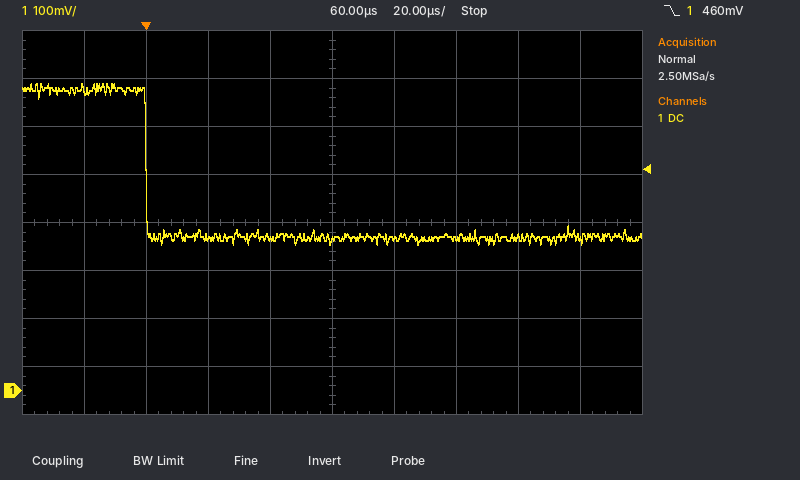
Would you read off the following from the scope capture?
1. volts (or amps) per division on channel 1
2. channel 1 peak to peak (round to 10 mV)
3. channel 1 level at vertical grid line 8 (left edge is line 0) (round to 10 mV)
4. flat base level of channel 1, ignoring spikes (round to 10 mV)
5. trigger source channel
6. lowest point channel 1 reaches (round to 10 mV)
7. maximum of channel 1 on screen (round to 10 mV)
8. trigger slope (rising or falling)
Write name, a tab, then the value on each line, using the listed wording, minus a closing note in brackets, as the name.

volts (or amps) per division on channel 1	100 mV
channel 1 peak to peak	340 mV
channel 1 level at vertical grid line 8 (left edge is line 0)	320 mV
flat base level of channel 1, ignoring spikes	320 mV
trigger source channel	channel 1
lowest point channel 1 reaches	300 mV
maximum of channel 1 on screen	640 mV
trigger slope	falling
